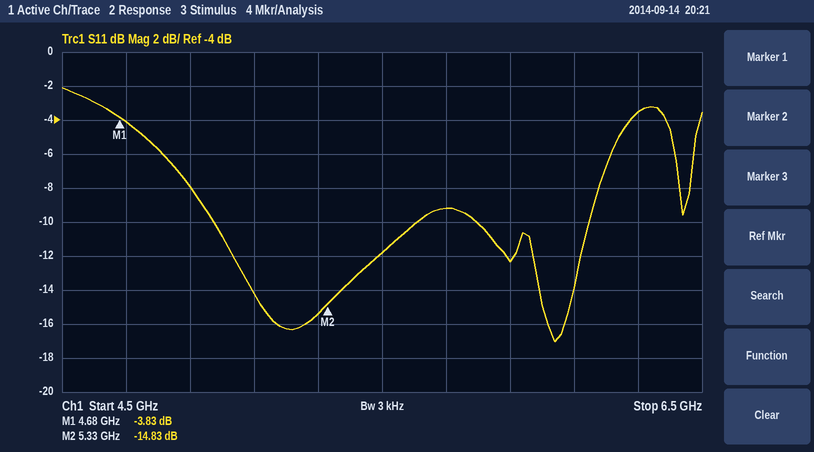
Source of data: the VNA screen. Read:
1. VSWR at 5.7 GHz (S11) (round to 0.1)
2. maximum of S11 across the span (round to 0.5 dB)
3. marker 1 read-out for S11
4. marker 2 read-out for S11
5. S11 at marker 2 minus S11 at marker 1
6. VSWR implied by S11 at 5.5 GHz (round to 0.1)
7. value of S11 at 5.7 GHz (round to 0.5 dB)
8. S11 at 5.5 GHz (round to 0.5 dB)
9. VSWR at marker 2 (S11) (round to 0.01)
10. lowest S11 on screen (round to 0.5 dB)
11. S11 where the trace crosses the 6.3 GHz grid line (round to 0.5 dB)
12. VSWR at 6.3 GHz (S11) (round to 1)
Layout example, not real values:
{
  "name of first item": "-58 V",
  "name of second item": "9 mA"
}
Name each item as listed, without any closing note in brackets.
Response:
{
  "VSWR at 5.7 GHz (S11)": "2.1",
  "maximum of S11 across the span": "-2.0 dB",
  "marker 1 read-out for S11": "-3.83 dB",
  "marker 2 read-out for S11": "-14.83 dB",
  "S11 at marker 2 minus S11 at marker 1": "-11.00 dB",
  "VSWR implied by S11 at 5.5 GHz": "1.7",
  "value of S11 at 5.7 GHz": "-9.0 dB",
  "S11 at 5.5 GHz": "-12.0 dB",
  "VSWR at marker 2 (S11)": "1.44",
  "lowest S11 on screen": "-17.0 dB",
  "S11 where the trace crosses the 6.3 GHz grid line": "-3.5 dB",
  "VSWR at 6.3 GHz (S11)": "5"
}
